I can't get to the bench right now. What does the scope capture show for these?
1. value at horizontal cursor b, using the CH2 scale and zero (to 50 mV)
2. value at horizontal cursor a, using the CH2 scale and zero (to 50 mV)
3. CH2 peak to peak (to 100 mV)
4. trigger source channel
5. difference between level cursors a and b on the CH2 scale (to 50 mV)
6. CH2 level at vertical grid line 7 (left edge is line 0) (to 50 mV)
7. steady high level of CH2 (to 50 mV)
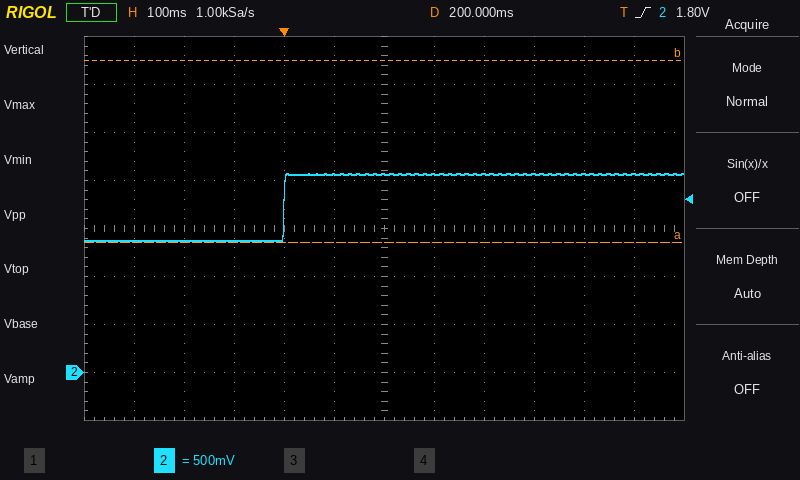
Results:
3.25 V
1.35 V
700 mV
CH2
1.90 V
2.05 V
2.05 V
